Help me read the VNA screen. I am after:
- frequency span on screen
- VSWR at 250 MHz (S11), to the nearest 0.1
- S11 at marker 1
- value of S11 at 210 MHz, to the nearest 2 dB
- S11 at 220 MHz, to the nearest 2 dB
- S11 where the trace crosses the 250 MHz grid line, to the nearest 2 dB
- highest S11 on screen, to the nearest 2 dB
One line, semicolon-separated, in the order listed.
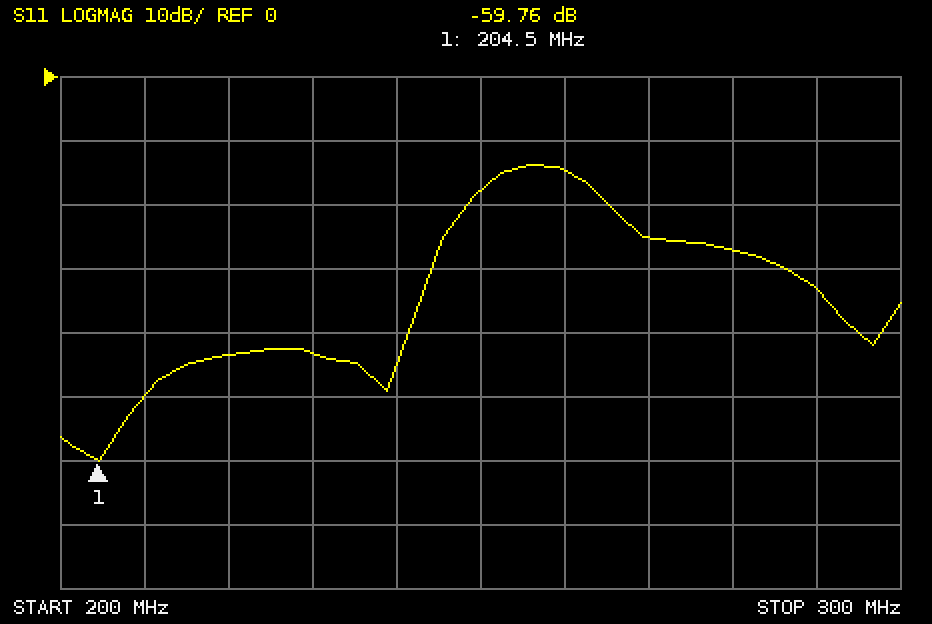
100 MHz; 1.3; -59.76 dB; -50 dB; -44 dB; -18 dB; -14 dB
